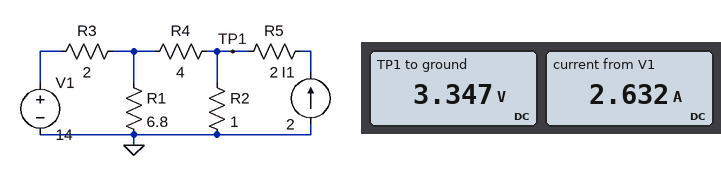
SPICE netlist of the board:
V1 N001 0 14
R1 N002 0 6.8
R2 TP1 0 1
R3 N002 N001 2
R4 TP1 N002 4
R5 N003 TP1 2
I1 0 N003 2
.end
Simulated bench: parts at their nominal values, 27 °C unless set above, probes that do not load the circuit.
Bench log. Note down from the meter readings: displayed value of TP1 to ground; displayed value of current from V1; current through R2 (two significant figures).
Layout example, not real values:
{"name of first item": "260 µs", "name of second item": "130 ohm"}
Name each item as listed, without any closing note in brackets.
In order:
{"displayed value of TP1 to ground": "3.347 V", "displayed value of current from V1": "2.632 A", "current through R2": "3.3 A"}
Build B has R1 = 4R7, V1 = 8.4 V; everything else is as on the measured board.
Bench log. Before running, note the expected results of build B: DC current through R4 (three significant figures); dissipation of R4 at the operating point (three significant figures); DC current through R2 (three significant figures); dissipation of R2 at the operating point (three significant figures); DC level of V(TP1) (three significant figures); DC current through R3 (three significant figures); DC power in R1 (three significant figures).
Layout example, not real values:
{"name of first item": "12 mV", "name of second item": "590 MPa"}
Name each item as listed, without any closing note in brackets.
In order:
{"DC current through R4": "608 mA", "dissipation of R4 at the operating point": "1.48 W", "DC current through R2": "2.61 A", "dissipation of R2 at the operating point": "6.80 W", "DC level of V(TP1)": "2.61 V", "DC current through R3": "1.68 A", "DC power in R1": "5.40 W"}
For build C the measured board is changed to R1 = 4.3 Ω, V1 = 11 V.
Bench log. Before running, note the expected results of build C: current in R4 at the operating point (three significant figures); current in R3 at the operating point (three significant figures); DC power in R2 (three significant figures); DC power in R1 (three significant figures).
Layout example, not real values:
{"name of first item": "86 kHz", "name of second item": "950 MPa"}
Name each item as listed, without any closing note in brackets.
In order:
{"current in R4 at the operating point": "865 mA", "current in R3 at the operating point": "2.34 A", "DC power in R2": "8.21 W", "DC power in R1": "9.31 W"}
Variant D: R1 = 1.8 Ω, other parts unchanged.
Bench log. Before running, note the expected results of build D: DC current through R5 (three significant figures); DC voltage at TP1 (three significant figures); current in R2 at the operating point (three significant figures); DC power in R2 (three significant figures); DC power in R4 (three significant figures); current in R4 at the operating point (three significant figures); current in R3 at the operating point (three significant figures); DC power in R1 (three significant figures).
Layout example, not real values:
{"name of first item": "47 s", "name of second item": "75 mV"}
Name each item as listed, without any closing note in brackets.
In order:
{"DC current through R5": "2.00 A", "DC voltage at TP1": "2.78 V", "current in R2 at the operating point": "2.78 A", "DC power in R2": "7.72 W", "DC power in R4": "2.43 W", "current in R4 at the operating point": "779 mA", "current in R3 at the operating point": "4.05 A", "DC power in R1": "19.3 W"}
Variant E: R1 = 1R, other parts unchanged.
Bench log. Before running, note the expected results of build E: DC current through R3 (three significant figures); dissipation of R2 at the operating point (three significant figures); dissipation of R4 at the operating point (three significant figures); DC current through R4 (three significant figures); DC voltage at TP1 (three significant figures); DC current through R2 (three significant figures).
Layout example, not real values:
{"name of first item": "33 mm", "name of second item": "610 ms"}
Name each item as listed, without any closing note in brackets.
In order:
{"DC current through R3": "4.82 A", "dissipation of R2 at the operating point": "6.10 W", "dissipation of R4 at the operating point": "886 mW", "DC current through R4": "471 mA", "DC voltage at TP1": "2.47 V", "DC current through R2": "2.47 A"}
